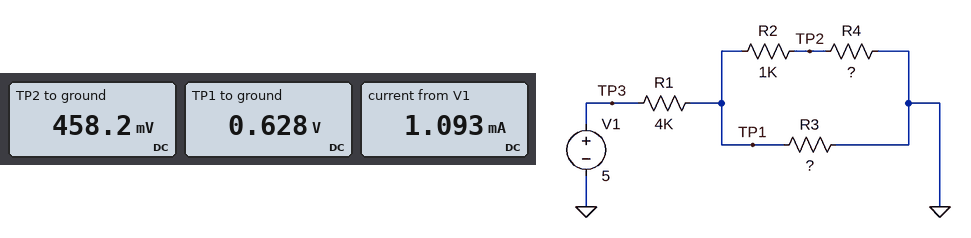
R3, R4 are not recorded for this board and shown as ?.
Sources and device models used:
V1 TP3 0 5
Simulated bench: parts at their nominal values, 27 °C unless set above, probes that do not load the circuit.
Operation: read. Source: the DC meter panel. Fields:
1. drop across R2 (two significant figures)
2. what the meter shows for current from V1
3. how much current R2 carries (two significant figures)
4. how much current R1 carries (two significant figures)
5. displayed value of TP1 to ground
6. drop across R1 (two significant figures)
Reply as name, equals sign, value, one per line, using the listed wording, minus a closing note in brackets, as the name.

drop across R2 = 170 mV
what the meter shows for current from V1 = 1.093 mA
how much current R2 carries = 170 µA
how much current R1 carries = 1.1 mA
displayed value of TP1 to ground = 0.628 V
drop across R1 = 4.4 V
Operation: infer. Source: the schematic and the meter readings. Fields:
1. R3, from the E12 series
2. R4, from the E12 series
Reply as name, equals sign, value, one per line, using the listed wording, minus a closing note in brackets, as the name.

R3, from the E12 series = 680 Ω
R4, from the E12 series = 2.7 kΩ
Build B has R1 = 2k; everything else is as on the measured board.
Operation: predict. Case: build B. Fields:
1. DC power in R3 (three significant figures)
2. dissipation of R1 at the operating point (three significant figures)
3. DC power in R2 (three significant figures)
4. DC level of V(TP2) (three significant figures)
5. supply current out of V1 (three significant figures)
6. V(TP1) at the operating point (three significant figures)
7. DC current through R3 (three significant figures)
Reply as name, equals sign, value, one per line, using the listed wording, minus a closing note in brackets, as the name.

DC power in R3 = 1.83 mW
dissipation of R1 at the operating point = 7.54 mW
DC power in R2 = 90.9 µW
DC level of V(TP2) = 814 mV
supply current out of V1 = 1.94 mA
V(TP1) at the operating point = 1.12 V
DC current through R3 = 1.64 mA
